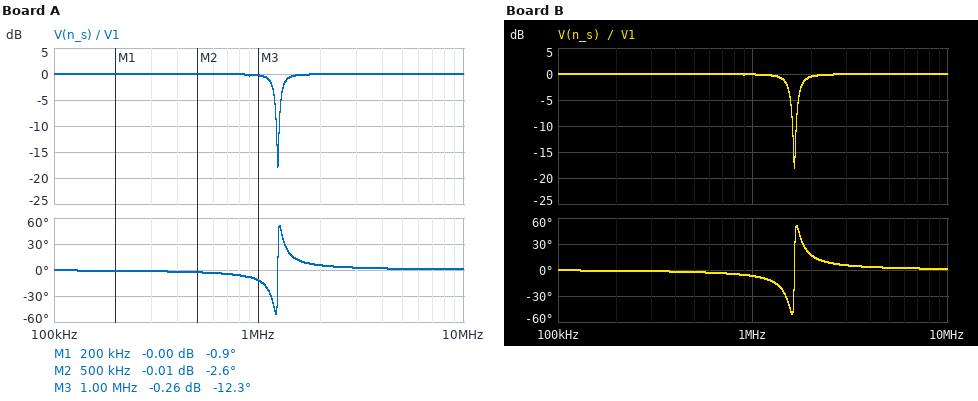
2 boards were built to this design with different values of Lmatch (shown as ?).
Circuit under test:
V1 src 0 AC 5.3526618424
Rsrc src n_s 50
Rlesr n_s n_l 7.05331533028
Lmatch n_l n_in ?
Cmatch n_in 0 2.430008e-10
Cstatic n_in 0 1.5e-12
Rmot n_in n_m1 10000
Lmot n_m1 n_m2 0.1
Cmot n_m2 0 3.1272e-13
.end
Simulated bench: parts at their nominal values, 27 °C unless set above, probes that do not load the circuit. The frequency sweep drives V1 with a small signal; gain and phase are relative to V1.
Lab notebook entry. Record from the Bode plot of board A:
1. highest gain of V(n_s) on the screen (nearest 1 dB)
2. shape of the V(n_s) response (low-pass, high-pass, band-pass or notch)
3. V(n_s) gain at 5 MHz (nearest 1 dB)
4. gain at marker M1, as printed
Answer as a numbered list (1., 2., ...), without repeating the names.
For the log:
1. 0 dB
2. notch
3. 0 dB
4. -0.00 dB
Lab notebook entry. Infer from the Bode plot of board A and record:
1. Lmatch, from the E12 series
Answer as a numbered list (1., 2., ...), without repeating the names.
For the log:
1. 68 µH
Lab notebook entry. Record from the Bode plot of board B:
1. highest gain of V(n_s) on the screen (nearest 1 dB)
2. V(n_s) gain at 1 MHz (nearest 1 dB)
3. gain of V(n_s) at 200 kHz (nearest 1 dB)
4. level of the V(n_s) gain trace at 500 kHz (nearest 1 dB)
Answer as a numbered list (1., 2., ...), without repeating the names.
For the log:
1. 0 dB
2. 0 dB
3. 0 dB
4. 0 dB
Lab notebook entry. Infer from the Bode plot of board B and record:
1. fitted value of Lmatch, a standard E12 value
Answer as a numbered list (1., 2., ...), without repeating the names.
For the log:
1. 39 µH
